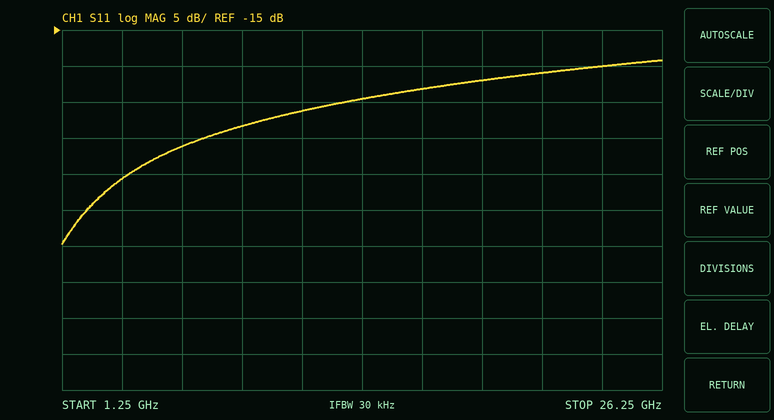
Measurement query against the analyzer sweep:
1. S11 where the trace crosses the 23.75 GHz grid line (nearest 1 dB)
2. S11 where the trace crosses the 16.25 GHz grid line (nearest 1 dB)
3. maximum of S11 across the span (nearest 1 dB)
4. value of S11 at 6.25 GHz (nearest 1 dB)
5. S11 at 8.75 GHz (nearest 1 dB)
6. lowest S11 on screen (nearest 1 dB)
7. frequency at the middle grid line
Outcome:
-20 dB
-23 dB
-19 dB
-31 dB
-28 dB
-45 dB
13.75 GHz
